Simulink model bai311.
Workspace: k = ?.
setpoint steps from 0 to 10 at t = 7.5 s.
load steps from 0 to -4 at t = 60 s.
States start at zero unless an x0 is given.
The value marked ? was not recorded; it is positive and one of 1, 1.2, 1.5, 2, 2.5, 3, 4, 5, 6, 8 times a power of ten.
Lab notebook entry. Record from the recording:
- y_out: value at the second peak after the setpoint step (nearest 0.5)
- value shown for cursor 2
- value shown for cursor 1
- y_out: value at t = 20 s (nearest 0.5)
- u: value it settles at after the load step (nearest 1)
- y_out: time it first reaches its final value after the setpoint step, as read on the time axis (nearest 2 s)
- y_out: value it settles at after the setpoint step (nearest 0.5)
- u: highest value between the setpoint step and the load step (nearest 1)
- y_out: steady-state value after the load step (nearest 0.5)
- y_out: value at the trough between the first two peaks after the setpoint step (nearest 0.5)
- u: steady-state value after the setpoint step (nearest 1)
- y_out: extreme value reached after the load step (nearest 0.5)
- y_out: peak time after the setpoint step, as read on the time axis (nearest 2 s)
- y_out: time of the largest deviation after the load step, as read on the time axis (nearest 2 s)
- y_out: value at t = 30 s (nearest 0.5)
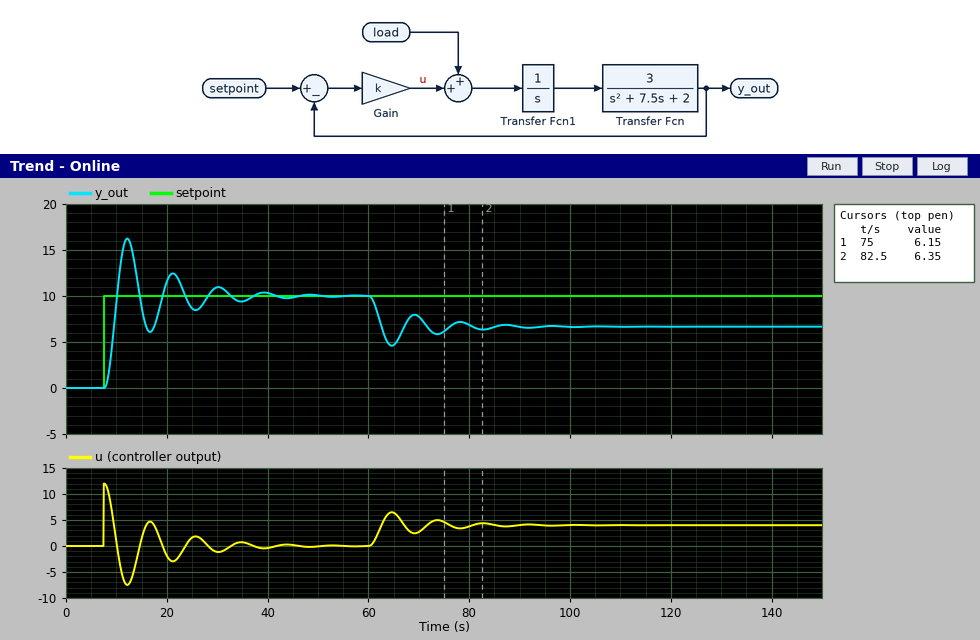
12.5
6.35
6.15
11.5
4
10 s
10.0
12
6.5
6.0
0
4.5
12 s
64 s
11.0
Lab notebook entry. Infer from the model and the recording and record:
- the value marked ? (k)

1.2
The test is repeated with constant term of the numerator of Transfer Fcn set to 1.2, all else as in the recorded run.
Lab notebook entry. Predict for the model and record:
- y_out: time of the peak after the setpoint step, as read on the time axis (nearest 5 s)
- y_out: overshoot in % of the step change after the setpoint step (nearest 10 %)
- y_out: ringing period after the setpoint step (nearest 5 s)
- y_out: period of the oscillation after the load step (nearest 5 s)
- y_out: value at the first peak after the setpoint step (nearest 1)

15 s
40 %
15 s
15 s
14
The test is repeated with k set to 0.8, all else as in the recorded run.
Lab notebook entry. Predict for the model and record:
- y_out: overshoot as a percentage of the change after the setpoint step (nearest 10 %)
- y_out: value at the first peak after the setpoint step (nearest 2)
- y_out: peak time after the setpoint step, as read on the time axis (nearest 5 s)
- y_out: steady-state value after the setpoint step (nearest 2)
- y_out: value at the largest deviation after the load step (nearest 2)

50 %
16
15 s
10
2
